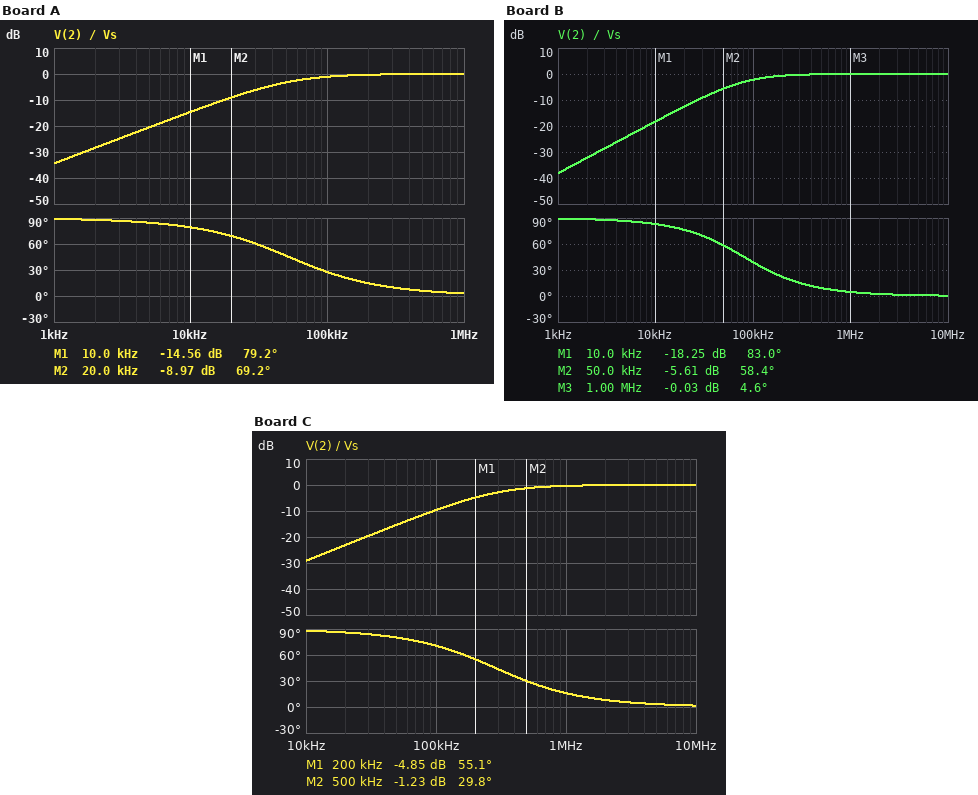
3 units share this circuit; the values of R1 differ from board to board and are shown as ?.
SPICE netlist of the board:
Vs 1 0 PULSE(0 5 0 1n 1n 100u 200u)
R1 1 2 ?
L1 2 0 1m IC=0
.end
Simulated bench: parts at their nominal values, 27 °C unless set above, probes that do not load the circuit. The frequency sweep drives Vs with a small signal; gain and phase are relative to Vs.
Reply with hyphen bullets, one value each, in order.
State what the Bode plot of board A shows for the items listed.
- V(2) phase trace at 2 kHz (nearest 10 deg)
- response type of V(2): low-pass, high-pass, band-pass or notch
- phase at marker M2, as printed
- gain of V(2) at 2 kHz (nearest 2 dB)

- 90 deg
- high-pass
- 69.2 deg
- -28 dB
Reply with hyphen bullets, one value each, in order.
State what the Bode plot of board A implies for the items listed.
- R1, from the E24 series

- 330 Ω
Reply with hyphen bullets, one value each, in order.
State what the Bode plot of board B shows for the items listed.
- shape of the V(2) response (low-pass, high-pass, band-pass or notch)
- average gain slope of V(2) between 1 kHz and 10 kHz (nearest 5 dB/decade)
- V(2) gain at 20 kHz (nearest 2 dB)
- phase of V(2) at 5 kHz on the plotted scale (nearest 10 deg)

- high-pass
- 20 dB/decade
- -12 dB
- 90 deg
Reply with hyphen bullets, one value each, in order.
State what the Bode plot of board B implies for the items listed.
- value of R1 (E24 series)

- 510 Ω
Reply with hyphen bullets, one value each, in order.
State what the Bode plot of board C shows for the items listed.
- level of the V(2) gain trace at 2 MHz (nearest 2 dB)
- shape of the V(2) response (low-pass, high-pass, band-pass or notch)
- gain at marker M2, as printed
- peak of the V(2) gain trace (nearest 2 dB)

- 0 dB
- high-pass
- -1.23 dB
- 0 dB
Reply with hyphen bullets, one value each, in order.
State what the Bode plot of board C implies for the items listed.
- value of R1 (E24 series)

- 1.8 kΩ
